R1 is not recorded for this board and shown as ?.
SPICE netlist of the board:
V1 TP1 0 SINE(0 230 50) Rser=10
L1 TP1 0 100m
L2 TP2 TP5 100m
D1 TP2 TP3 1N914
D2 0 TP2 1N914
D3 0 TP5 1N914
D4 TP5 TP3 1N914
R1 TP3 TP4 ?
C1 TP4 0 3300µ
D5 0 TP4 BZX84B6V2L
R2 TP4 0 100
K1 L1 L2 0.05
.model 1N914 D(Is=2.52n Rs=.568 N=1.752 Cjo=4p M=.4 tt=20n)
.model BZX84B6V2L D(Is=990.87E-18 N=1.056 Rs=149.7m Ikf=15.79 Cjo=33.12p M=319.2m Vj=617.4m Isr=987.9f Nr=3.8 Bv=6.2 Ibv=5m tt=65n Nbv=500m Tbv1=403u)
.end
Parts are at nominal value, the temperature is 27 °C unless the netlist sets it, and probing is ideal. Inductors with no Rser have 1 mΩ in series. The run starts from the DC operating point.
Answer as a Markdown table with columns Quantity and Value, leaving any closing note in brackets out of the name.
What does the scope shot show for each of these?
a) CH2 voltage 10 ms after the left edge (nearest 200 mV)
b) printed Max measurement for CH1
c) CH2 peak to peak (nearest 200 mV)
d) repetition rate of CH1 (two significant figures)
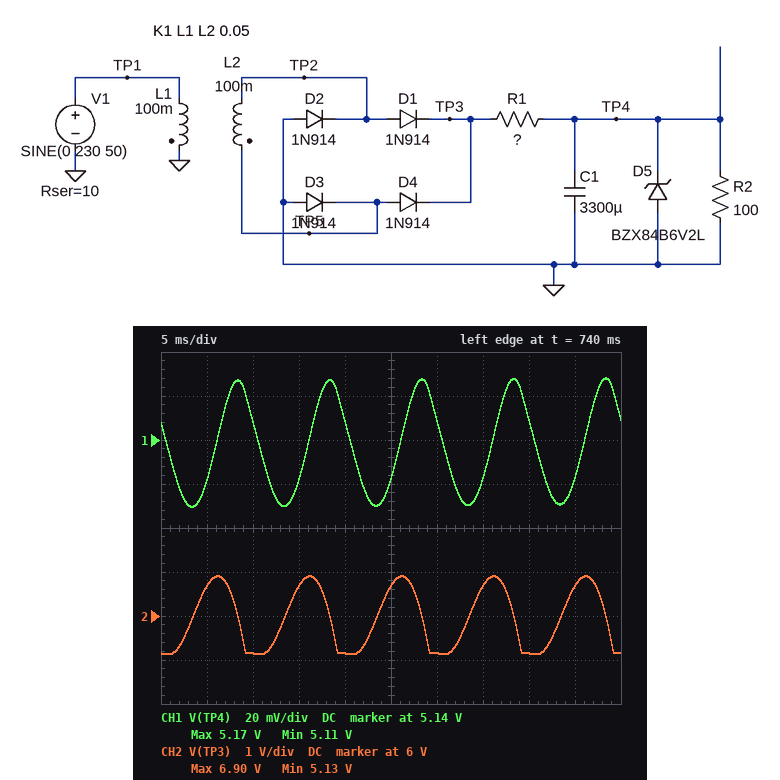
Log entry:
| Quantity | Value |
|---|---|
| CH2 voltage 10 ms after the left edge | 5.2 V |
| printed Max measurement for CH1 | 5.17 V |
| CH2 peak to peak | 1.8 V |
| repetition rate of CH1 | 100 Hz |
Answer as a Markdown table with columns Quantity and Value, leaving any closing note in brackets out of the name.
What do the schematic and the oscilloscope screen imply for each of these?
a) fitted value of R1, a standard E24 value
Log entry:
| Quantity | Value |
|---|---|
| fitted value of R1, a standard E24 value | 16 Ω |
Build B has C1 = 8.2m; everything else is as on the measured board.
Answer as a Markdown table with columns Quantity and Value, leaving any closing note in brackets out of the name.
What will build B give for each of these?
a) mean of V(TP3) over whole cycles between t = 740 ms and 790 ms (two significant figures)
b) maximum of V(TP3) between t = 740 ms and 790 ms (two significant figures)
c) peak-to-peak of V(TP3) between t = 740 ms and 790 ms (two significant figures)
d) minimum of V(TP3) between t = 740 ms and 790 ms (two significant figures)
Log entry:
| Quantity | Value |
|---|---|
| mean of V(TP3) over whole cycles between t = 740 ms and 790 ms | 5.8 V |
| maximum of V(TP3) between t = 740 ms and 790 ms | 6.8 V |
| peak-to-peak of V(TP3) between t = 740 ms and 790 ms | 1.9 V |
| minimum of V(TP3) between t = 740 ms and 790 ms | 4.9 V |
